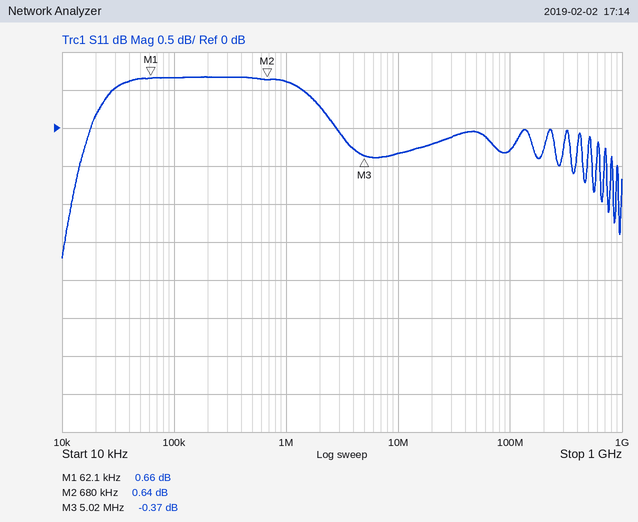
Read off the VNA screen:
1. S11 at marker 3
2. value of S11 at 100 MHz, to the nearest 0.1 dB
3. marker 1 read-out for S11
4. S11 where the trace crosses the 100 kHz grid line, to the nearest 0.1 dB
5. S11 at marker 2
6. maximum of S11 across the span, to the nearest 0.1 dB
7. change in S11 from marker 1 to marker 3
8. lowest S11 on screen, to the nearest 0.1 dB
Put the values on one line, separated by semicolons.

-0.37 dB; -0.3 dB; 0.66 dB; 0.7 dB; 0.64 dB; 0.7 dB; -1.03 dB; -1.7 dB
